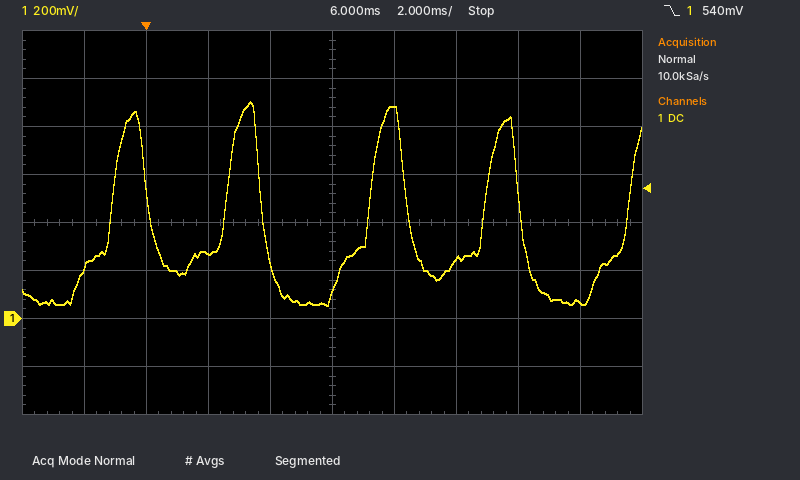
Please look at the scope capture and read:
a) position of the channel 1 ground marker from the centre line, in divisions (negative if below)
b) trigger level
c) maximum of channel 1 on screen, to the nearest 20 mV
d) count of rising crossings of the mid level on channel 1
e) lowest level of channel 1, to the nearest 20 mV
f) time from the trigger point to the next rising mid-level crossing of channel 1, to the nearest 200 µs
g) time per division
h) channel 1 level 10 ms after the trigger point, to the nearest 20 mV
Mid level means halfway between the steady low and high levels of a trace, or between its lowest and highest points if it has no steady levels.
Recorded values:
-2.0 div
540 mV
900 mV
5
60 mV
2.6 ms
2 ms
240 mV
